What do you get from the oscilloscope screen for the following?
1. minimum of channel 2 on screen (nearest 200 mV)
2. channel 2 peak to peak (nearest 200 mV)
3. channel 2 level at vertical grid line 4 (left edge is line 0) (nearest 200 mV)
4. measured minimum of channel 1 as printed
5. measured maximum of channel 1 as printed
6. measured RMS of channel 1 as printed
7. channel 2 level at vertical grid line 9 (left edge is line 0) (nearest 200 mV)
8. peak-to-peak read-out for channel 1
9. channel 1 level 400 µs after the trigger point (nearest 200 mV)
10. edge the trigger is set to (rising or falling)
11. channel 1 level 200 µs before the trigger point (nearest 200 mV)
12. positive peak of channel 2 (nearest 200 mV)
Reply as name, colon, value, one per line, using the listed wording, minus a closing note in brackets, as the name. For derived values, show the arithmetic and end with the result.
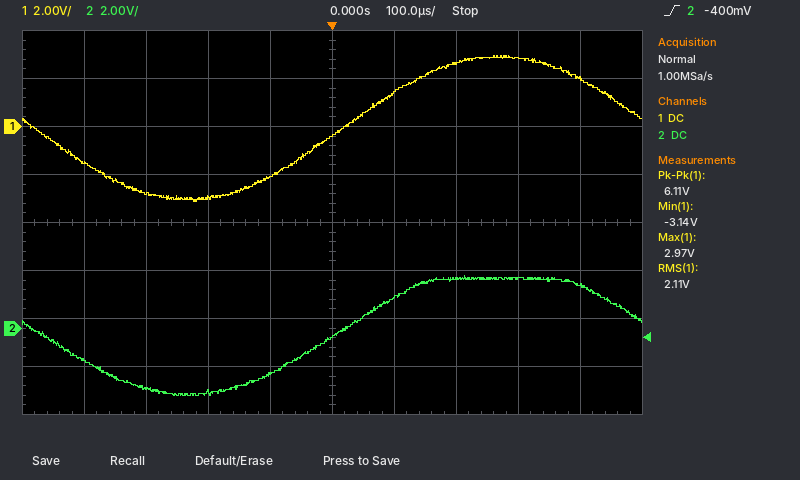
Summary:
minimum of channel 2 on screen: -2.8 V
channel 2 peak to peak: 2.2 V − (-2.8 V) = 5.0 V
channel 2 level at vertical grid line 4 (left edge is line 0): -2.0 V
measured minimum of channel 1 as printed: -3.14 V
measured maximum of channel 1 as printed: 2.97 V
measured RMS of channel 1 as printed: 2.11 V
channel 2 level at vertical grid line 9 (left edge is line 0): 1.8 V
peak-to-peak read-out for channel 1: 6.11 V
channel 1 level 400 µs after the trigger point: 2.0 V
edge the trigger is set to: rising
channel 1 level 200 µs before the trigger point: -3.0 V
positive peak of channel 2: 2.2 V
